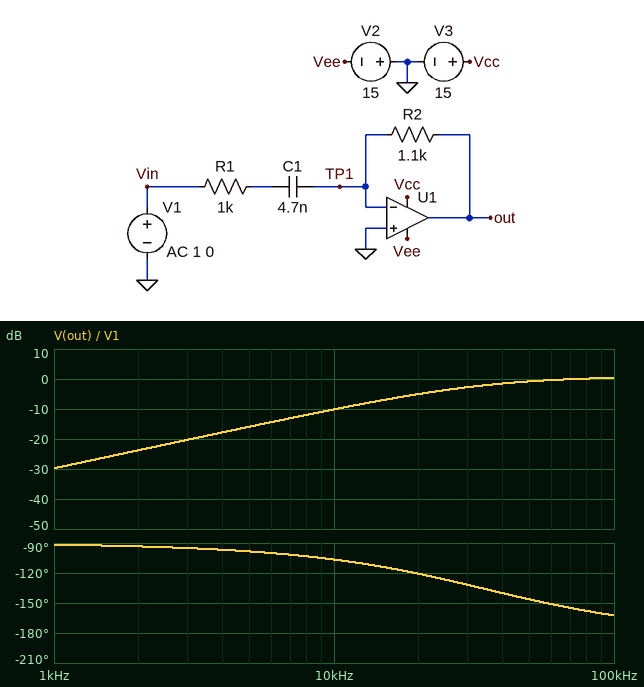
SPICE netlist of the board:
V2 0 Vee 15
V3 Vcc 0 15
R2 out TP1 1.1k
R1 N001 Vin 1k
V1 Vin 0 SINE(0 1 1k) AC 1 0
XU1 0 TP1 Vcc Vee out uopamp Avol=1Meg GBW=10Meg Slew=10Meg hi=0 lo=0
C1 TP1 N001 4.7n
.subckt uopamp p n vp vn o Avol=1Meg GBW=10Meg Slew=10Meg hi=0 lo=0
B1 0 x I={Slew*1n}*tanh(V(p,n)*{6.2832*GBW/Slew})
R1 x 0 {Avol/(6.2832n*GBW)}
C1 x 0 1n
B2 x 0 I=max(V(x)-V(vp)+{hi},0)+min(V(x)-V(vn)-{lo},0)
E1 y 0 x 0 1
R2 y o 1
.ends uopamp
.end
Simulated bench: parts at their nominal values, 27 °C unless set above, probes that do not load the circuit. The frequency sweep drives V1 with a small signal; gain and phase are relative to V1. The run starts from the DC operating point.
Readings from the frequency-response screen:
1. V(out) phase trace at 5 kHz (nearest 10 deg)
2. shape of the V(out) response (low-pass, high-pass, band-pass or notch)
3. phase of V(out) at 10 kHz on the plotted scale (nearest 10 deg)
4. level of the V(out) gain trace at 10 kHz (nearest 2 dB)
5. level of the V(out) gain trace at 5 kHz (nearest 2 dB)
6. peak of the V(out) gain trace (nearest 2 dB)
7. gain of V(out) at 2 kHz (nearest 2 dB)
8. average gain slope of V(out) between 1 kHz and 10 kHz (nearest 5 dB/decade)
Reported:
-100 deg
high-pass
-110 deg
-10 dB
-16 dB
0 dB
-24 dB
20 dB/decade
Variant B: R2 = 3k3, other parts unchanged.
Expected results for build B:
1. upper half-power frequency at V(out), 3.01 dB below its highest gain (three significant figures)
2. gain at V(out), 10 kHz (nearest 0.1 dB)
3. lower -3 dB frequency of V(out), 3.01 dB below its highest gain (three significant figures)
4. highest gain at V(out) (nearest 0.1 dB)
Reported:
2.37 MHz
-0.6 dB
33.3 kHz
10.3 dB
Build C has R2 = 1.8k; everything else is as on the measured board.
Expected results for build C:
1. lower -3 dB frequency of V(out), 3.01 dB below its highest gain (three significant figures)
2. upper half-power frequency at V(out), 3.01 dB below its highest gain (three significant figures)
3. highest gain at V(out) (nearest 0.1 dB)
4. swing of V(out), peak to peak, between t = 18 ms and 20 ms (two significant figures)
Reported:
33.4 kHz
3.62 MHz
5.1 dB
110 mV
